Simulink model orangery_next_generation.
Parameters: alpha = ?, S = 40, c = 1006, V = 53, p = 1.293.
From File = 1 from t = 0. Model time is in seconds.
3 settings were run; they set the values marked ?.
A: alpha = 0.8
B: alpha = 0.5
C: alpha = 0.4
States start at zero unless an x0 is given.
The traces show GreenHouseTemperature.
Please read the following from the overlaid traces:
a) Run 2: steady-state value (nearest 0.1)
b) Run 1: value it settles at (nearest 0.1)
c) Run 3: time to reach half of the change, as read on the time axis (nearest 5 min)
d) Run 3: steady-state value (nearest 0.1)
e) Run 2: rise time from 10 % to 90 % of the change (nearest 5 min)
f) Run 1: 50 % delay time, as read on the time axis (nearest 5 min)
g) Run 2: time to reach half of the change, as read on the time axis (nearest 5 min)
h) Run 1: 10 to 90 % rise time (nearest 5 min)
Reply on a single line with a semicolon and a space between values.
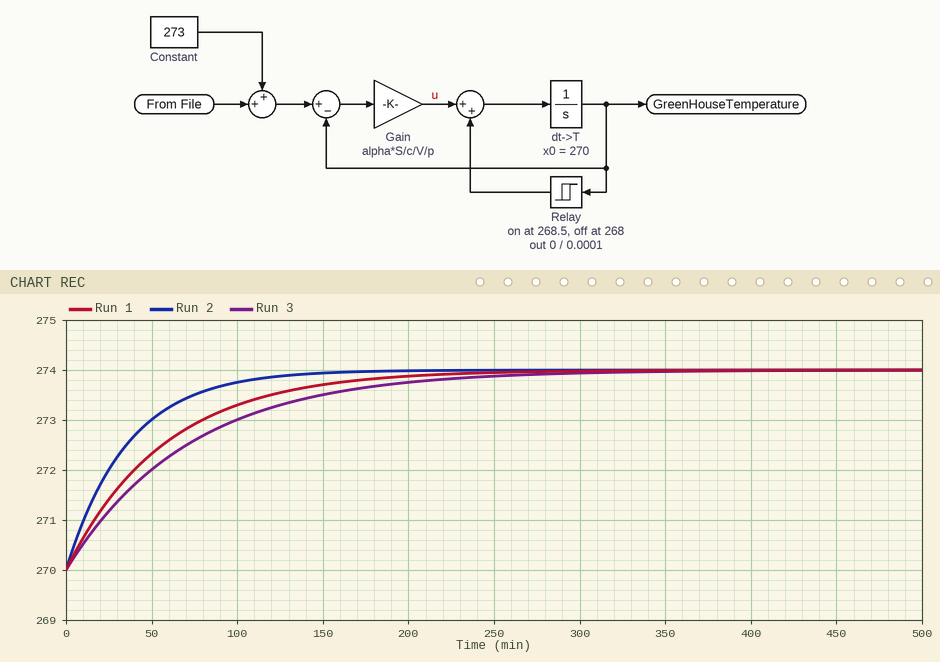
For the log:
274.0; 274.0; 50 min; 274.0; 80 min; 40 min; 25 min; 125 min
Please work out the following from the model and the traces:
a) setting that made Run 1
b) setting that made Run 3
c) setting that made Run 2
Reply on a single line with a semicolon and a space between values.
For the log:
B; C; A
